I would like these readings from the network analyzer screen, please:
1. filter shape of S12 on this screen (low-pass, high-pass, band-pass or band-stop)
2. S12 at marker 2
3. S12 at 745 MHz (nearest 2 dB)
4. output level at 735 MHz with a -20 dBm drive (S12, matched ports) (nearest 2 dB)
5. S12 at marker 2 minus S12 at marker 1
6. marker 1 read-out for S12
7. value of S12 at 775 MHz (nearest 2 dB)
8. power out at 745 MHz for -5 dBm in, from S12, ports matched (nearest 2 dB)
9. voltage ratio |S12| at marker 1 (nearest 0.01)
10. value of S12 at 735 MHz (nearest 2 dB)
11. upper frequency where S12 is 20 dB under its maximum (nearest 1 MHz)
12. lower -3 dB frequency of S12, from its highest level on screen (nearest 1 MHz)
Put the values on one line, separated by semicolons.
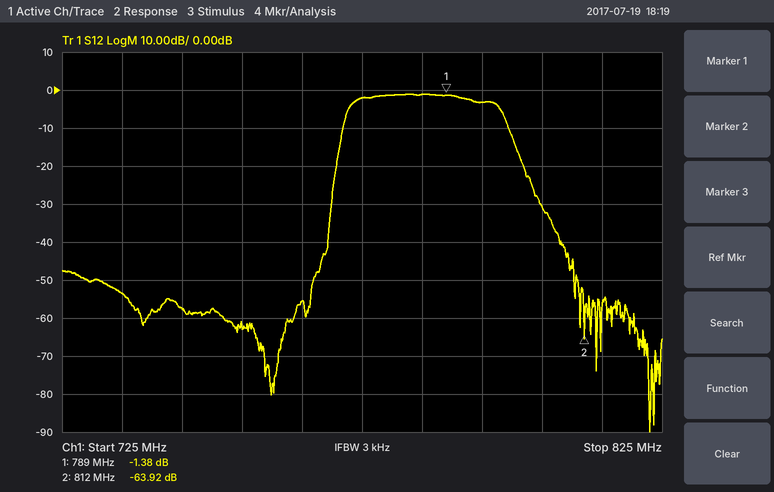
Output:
band-pass; -63.92 dB; -58 dB; -74 dBm; -62.54 dB; -1.38 dB; -2 dB; -62 dBm; 0.85; -54 dB; 802 MHz; 773 MHz
